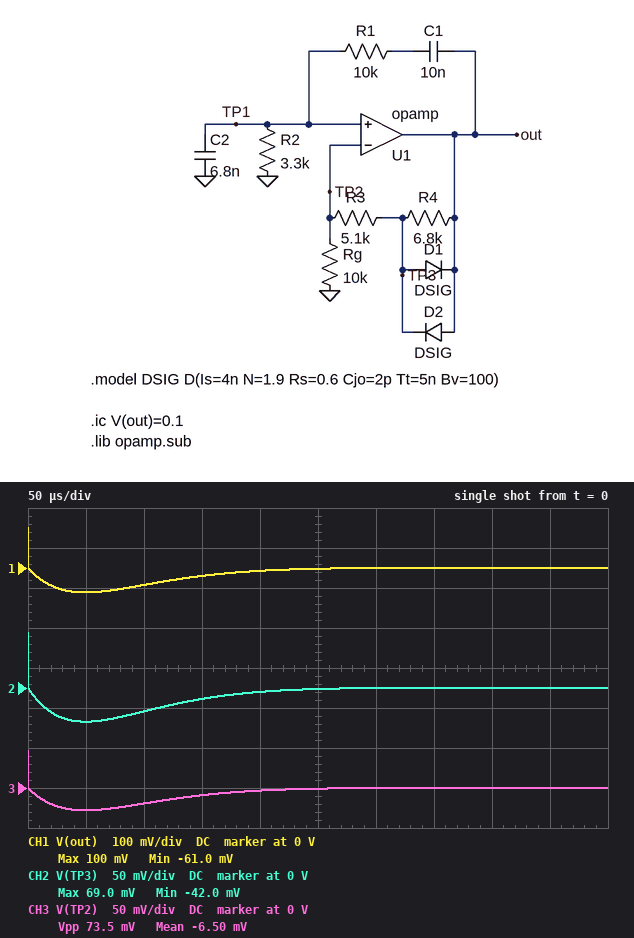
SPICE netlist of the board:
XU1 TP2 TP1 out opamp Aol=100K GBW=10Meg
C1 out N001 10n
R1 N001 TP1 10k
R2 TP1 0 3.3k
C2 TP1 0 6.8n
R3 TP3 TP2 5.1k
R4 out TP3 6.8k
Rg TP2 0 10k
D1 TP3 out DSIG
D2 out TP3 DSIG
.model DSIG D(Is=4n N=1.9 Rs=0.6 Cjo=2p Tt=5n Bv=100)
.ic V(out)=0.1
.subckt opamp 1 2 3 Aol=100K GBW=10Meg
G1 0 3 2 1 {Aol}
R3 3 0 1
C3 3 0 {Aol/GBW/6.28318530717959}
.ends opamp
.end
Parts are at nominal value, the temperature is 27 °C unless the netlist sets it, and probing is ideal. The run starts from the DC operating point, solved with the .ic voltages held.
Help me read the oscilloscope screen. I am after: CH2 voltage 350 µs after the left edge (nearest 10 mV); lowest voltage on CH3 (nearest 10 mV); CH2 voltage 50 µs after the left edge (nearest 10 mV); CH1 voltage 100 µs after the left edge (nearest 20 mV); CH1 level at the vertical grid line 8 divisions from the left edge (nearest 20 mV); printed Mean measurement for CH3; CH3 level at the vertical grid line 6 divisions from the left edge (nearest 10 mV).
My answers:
0 V
-30 mV
-40 mV
-40 mV
0 V
-6.50 mV
0 V
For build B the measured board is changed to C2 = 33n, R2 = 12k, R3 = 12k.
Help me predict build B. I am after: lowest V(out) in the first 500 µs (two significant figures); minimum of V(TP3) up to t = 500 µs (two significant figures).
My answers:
-81 mV
-62 mV
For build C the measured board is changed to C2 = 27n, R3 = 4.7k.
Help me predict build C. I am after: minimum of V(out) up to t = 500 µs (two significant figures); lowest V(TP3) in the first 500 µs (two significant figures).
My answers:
-32 mV
-22 mV
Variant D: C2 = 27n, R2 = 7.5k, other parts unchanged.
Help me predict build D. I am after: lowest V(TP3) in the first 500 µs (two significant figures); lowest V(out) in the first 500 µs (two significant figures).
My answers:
-35 mV
-51 mV
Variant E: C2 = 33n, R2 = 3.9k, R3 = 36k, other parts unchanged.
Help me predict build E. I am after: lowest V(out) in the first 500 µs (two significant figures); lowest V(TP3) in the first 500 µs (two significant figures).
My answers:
-130 mV
-110 mV
